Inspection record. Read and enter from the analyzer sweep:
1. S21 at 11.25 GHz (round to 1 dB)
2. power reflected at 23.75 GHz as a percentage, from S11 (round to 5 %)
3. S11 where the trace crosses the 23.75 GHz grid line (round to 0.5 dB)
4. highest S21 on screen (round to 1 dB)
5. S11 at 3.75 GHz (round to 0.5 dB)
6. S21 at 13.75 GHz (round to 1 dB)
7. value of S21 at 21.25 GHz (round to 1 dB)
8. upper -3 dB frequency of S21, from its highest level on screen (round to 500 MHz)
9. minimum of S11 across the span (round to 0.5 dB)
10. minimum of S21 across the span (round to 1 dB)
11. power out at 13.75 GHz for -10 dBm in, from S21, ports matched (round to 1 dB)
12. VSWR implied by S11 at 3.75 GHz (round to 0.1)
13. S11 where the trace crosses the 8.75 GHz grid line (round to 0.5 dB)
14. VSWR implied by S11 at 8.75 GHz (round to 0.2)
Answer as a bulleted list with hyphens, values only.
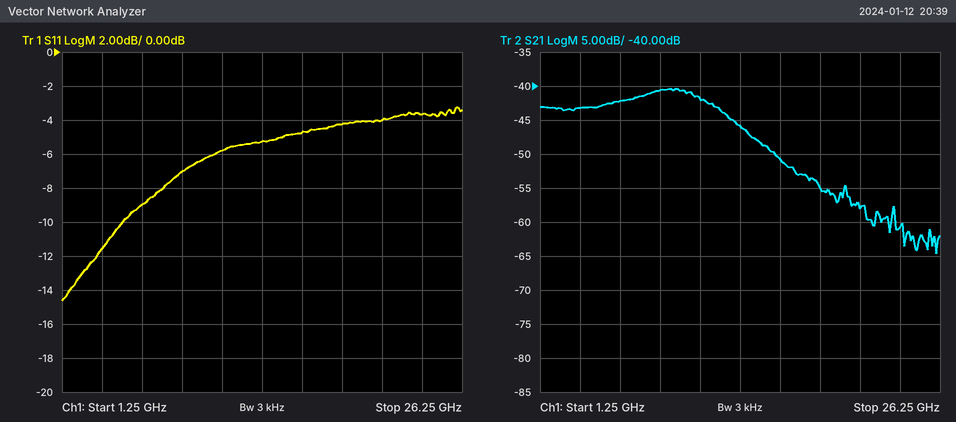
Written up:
- -42 dB
- 45 %
- -3.5 dB
- -40 dB
- -11.5 dB
- -46 dB
- -58 dB
- 12.5 GHz
- -14.5 dB
- -65 dB
- -56 dBm
- 1.7
- -7.0 dB
- 2.6
